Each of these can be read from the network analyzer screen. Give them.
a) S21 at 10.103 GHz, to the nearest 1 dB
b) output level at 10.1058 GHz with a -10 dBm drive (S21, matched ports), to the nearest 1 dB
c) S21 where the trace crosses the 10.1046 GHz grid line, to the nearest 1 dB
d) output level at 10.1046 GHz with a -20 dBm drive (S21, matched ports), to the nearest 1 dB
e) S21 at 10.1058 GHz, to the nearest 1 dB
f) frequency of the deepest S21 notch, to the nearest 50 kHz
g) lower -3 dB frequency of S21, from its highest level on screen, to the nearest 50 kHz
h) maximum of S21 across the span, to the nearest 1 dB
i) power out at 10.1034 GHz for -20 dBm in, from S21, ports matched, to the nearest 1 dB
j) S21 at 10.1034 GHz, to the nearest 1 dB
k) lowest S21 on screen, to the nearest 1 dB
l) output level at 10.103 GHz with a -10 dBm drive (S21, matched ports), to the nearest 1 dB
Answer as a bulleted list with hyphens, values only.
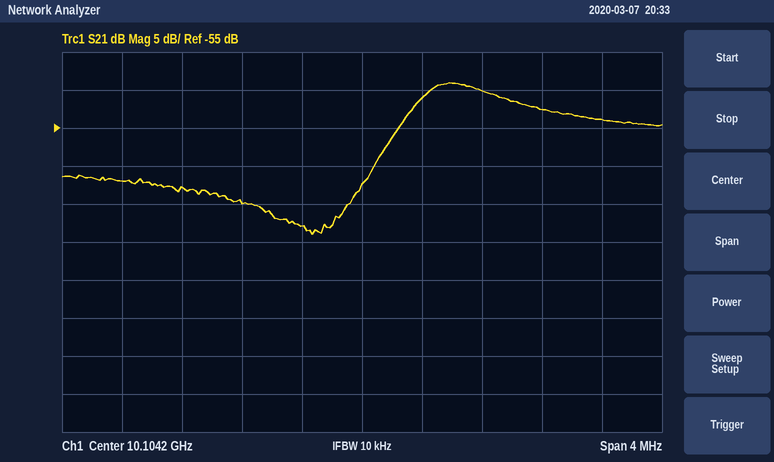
- -63 dB
- -64 dBm
- -51 dB
- -71 dBm
- -54 dB
- 10.10385 GHz
- 10.10455 GHz
- -49 dB
- -85 dBm
- -65 dB
- -69 dB
- -73 dBm
